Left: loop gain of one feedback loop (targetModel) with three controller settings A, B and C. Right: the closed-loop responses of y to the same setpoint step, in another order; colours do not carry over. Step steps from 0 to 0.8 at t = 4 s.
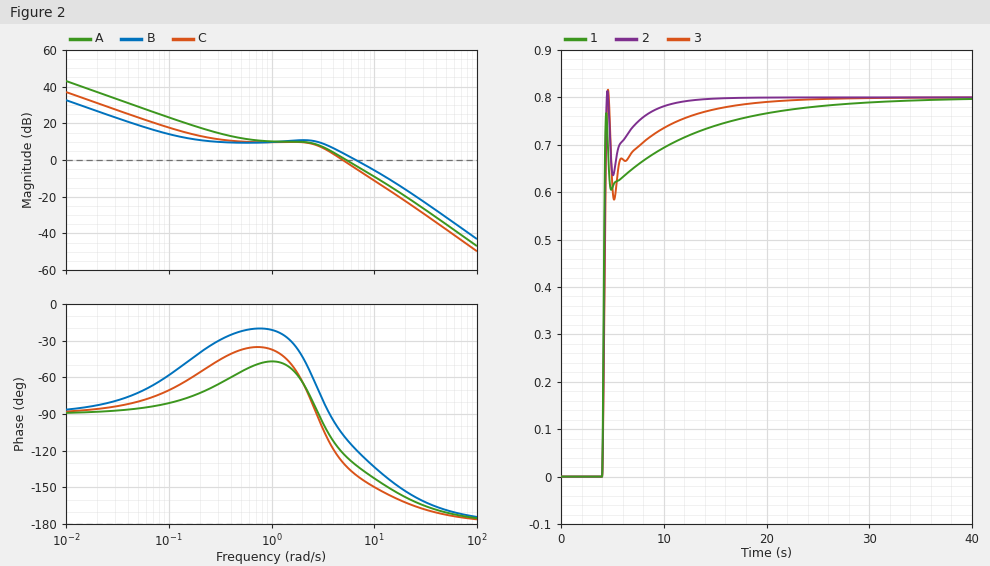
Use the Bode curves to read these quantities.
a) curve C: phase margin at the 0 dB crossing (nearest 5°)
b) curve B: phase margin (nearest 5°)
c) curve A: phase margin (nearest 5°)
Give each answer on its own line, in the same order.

50°
60°
55°
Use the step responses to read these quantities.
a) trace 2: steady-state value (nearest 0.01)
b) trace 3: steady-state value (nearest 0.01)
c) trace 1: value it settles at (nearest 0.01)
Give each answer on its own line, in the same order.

0.80
0.80
0.80
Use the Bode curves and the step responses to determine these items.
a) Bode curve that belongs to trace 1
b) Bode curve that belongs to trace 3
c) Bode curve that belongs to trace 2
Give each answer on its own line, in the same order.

B
C
A
